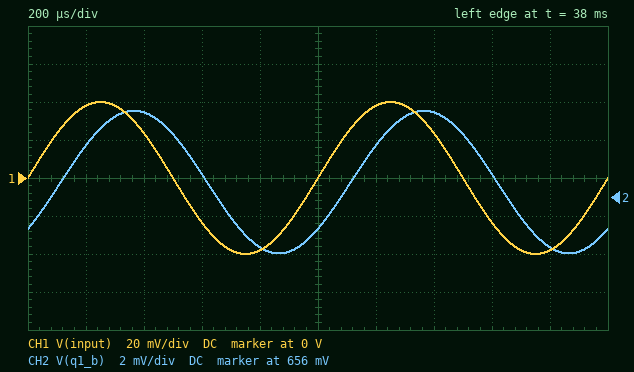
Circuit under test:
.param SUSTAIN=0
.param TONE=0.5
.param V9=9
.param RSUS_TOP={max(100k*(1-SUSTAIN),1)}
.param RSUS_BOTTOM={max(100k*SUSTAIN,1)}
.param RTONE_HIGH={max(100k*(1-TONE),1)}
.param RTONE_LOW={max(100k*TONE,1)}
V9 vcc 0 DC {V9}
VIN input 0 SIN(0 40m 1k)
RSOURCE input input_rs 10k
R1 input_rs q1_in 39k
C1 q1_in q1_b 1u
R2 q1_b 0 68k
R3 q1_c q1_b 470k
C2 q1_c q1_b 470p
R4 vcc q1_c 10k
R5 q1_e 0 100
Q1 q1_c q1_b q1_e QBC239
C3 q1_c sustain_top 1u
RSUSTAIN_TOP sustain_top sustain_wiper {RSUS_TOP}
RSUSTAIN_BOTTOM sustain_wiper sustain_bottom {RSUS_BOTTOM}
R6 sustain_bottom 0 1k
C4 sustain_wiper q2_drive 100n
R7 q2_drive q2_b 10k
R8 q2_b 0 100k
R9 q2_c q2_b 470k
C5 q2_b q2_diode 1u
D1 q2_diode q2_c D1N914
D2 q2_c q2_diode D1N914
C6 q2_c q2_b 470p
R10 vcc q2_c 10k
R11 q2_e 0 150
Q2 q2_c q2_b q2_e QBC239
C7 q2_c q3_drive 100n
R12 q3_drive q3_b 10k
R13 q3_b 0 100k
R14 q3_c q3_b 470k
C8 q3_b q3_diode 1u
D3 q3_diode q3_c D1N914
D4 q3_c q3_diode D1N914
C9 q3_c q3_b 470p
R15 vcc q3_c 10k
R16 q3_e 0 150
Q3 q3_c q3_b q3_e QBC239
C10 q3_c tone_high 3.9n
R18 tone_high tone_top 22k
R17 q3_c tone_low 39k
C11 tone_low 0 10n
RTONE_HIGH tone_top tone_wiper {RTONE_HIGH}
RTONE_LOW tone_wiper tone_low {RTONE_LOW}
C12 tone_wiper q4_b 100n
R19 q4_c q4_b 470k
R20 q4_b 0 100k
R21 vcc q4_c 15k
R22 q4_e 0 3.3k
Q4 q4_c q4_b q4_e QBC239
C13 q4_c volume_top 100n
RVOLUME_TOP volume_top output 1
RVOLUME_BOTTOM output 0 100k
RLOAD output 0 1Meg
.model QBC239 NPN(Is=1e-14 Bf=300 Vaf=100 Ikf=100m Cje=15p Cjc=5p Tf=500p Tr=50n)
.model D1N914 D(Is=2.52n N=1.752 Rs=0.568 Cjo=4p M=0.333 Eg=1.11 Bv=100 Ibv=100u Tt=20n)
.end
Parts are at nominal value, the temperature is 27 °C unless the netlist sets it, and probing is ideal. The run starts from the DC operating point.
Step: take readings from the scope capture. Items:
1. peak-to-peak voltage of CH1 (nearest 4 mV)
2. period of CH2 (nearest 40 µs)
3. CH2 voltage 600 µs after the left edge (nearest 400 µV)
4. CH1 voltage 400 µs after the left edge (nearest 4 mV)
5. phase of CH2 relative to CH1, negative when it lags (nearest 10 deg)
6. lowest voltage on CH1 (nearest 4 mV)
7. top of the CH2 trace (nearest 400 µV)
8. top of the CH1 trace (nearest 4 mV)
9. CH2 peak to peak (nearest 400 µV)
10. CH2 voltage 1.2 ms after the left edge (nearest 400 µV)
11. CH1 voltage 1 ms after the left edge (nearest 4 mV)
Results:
80 mV
1.00 ms
657.2 mV
24 mV
-40 deg
-40 mV
660.4 mV
40 mV
7.6 mV
658.8 mV
0 V
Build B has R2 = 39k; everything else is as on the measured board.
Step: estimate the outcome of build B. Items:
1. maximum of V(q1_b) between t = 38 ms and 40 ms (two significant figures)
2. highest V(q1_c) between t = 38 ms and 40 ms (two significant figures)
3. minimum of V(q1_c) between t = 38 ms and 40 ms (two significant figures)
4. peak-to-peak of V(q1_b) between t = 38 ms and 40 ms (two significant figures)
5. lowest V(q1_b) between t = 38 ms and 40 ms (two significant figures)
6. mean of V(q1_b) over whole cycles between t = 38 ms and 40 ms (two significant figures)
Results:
610 mV
8.1 V
7.8 V
13 mV
590 mV
600 mV
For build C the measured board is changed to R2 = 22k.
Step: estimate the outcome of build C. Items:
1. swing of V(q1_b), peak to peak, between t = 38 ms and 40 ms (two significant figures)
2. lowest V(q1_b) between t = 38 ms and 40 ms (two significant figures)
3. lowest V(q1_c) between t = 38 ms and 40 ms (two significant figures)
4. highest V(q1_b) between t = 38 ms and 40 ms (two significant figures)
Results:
24 mV
380 mV
8.8 V
410 mV
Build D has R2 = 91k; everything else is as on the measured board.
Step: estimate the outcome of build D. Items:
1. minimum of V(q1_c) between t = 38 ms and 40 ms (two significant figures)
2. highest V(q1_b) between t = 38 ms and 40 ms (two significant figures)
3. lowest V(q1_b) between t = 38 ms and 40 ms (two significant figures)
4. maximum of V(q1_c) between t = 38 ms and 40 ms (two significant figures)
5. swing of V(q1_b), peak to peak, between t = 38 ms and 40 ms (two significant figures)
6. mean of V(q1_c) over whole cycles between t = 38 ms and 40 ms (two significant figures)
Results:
4.6 V
680 mV
670 mV
5.0 V
6.9 mV
4.8 V
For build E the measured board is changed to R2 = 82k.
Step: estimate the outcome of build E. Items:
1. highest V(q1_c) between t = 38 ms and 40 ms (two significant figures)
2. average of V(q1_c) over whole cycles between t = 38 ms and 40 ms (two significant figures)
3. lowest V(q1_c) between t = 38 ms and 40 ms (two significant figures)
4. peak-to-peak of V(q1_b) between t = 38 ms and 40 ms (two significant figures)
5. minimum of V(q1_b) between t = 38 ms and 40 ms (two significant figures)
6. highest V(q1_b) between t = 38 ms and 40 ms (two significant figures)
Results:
5.3 V
5.1 V
4.9 V
7.1 mV
660 mV
670 mV
